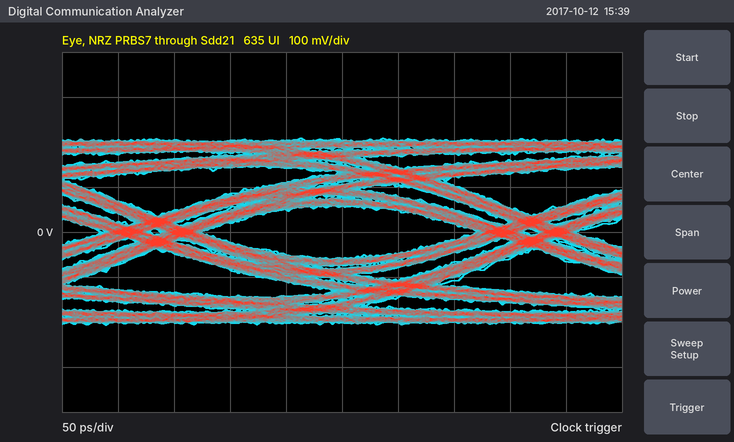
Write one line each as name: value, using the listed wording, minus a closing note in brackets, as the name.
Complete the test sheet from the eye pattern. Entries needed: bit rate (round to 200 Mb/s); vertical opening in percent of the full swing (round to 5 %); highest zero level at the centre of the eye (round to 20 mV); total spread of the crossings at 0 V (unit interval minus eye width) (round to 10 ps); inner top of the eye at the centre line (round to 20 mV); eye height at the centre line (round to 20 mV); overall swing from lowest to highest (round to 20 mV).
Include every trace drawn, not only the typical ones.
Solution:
bit rate: 3.0 Gb/s
vertical opening in percent of the full swing: 30 %
highest zero level at the centre of the eye: -60 mV
total spread of the crossings at 0 V (unit interval minus eye width): 90 ps
inner top of the eye at the centre line: 60 mV
eye height at the centre line: 120 mV
overall swing from lowest to highest: 420 mV
